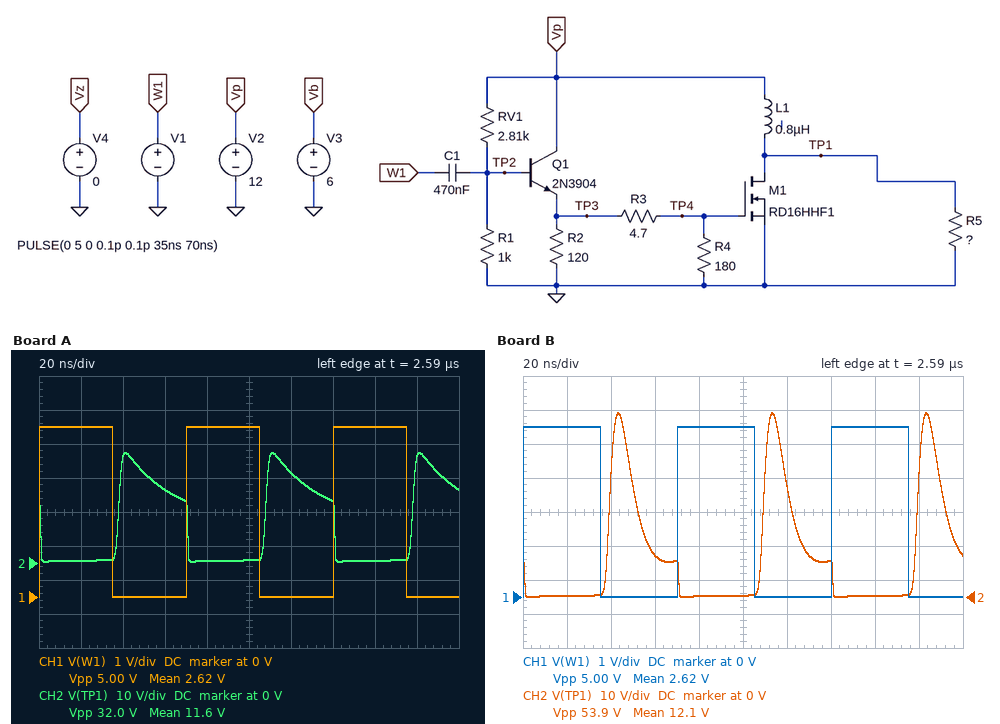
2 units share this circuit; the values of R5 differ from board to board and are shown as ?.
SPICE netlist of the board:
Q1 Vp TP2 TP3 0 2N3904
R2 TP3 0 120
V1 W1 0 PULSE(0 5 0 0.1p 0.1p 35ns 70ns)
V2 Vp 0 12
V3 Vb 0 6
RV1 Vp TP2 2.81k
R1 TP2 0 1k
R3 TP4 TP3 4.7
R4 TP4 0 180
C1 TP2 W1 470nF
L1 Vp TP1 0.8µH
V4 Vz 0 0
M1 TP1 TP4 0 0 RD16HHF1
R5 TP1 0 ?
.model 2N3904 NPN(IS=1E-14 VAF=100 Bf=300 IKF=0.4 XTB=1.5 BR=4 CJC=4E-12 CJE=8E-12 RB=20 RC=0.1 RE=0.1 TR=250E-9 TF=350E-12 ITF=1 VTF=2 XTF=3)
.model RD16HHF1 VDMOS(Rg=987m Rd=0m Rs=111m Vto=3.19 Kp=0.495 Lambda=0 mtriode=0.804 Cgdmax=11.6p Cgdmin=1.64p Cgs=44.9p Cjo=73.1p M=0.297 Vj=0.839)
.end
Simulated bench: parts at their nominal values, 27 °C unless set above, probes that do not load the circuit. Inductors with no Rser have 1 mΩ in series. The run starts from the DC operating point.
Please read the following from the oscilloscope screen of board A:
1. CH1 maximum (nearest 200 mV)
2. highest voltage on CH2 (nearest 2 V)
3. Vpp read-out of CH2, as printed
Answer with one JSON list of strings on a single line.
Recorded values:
["5.0 V", "32 V", "32.0 V"]
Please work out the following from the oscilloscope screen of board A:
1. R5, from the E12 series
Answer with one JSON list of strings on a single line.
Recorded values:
["33 Ω"]
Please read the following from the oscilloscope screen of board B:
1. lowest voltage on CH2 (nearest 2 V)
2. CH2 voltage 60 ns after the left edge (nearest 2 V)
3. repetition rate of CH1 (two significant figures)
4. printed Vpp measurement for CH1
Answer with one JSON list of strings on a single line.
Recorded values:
["0 V", "12 V", "14 MHz", "5.00 V"]
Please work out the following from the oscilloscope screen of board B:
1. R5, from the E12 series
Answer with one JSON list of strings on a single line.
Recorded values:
["120 Ω"]
